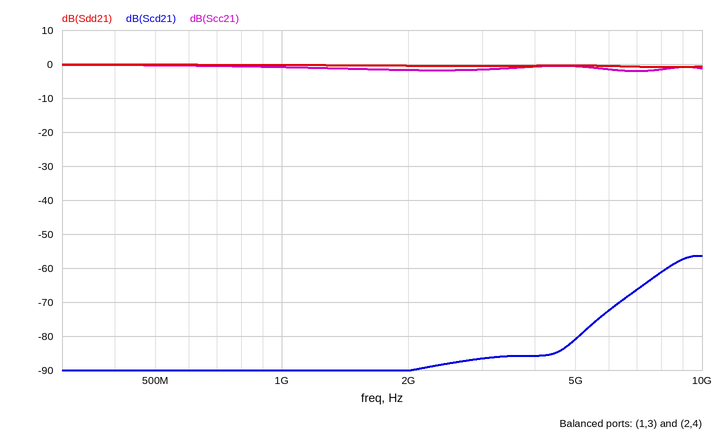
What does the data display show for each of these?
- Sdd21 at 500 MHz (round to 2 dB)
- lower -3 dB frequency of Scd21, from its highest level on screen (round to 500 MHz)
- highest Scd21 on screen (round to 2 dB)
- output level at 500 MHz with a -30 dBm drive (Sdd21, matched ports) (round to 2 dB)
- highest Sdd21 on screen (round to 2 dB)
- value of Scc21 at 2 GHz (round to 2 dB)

0 dB
8.5 GHz
-56 dB
-30 dBm
0 dB
-2 dB
